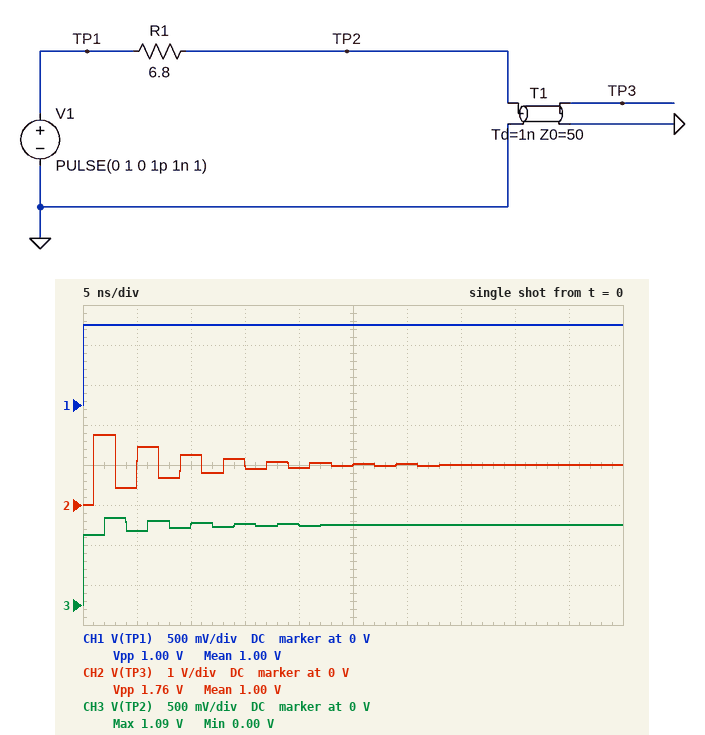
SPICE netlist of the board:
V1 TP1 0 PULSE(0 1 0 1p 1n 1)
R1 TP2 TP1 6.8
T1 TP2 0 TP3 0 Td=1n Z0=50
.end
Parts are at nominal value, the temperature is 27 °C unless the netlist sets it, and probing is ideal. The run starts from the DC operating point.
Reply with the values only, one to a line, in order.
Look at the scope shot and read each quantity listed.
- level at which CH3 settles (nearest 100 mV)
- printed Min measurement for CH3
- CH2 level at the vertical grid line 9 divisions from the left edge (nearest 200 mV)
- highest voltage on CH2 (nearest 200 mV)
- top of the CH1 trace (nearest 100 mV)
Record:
1.0 V
0.00 V
1.0 V
1.8 V
1.0 V
